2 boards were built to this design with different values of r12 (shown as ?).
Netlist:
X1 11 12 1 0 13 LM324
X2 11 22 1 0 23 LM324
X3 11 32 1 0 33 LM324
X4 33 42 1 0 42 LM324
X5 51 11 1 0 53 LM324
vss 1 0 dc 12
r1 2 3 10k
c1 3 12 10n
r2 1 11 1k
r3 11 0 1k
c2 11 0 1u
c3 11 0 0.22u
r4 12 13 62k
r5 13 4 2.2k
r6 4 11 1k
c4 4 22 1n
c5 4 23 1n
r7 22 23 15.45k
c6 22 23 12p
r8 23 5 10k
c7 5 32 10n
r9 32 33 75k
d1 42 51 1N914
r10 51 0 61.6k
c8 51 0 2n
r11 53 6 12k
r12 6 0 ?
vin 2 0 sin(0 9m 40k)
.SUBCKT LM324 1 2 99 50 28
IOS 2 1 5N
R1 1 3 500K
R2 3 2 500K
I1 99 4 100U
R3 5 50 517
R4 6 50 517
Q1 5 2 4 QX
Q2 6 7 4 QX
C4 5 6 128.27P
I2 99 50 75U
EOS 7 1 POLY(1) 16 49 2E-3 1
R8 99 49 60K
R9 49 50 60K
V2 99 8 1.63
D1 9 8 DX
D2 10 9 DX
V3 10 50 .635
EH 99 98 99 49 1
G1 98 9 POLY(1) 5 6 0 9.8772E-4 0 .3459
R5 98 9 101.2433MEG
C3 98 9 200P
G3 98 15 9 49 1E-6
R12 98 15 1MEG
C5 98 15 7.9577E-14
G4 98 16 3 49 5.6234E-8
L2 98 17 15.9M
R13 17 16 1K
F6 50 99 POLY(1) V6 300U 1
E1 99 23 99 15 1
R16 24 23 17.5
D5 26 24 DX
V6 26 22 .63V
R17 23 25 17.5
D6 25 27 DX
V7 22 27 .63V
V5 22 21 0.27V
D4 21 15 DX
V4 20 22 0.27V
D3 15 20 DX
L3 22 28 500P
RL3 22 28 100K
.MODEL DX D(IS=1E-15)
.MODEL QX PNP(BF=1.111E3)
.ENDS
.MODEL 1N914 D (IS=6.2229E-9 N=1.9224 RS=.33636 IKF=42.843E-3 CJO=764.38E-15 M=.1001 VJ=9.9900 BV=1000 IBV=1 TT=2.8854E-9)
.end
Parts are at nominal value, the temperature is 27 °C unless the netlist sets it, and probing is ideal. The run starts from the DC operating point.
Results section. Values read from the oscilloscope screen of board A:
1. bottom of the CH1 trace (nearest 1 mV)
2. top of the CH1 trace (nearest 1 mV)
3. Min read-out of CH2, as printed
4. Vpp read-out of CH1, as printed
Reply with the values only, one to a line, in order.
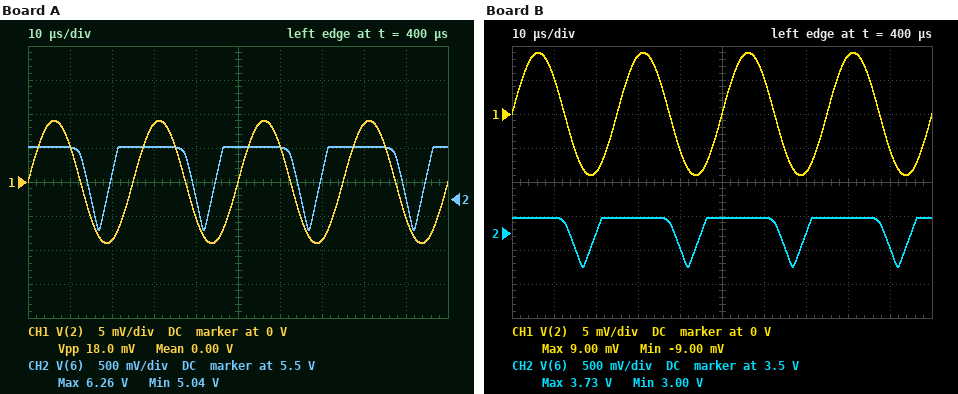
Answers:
-9 mV
9 mV
5.04 V
18.0 mV
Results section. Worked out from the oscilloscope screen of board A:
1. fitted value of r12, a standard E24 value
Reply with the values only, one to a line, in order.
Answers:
16 kΩ
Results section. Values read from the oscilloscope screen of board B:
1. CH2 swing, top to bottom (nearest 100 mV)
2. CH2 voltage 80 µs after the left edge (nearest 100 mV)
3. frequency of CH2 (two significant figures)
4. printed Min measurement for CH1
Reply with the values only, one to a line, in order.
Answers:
700 mV
3.7 V
40 kHz
-9.00 mV
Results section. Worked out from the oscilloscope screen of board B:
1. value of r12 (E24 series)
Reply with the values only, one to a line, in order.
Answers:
6.2 kΩ
